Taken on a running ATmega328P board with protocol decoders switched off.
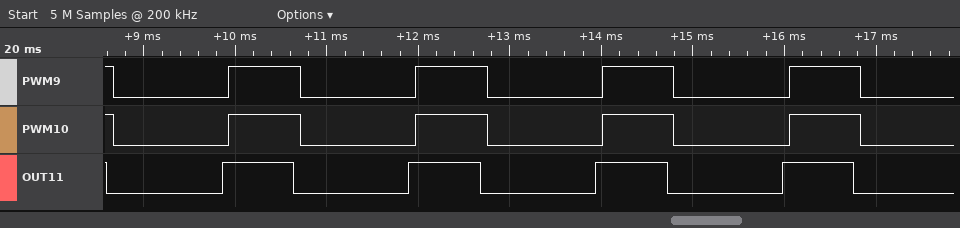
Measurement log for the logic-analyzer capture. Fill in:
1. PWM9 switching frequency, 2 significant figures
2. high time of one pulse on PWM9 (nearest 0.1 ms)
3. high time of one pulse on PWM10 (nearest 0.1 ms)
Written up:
490 Hz
0.8 ms
0.8 ms
